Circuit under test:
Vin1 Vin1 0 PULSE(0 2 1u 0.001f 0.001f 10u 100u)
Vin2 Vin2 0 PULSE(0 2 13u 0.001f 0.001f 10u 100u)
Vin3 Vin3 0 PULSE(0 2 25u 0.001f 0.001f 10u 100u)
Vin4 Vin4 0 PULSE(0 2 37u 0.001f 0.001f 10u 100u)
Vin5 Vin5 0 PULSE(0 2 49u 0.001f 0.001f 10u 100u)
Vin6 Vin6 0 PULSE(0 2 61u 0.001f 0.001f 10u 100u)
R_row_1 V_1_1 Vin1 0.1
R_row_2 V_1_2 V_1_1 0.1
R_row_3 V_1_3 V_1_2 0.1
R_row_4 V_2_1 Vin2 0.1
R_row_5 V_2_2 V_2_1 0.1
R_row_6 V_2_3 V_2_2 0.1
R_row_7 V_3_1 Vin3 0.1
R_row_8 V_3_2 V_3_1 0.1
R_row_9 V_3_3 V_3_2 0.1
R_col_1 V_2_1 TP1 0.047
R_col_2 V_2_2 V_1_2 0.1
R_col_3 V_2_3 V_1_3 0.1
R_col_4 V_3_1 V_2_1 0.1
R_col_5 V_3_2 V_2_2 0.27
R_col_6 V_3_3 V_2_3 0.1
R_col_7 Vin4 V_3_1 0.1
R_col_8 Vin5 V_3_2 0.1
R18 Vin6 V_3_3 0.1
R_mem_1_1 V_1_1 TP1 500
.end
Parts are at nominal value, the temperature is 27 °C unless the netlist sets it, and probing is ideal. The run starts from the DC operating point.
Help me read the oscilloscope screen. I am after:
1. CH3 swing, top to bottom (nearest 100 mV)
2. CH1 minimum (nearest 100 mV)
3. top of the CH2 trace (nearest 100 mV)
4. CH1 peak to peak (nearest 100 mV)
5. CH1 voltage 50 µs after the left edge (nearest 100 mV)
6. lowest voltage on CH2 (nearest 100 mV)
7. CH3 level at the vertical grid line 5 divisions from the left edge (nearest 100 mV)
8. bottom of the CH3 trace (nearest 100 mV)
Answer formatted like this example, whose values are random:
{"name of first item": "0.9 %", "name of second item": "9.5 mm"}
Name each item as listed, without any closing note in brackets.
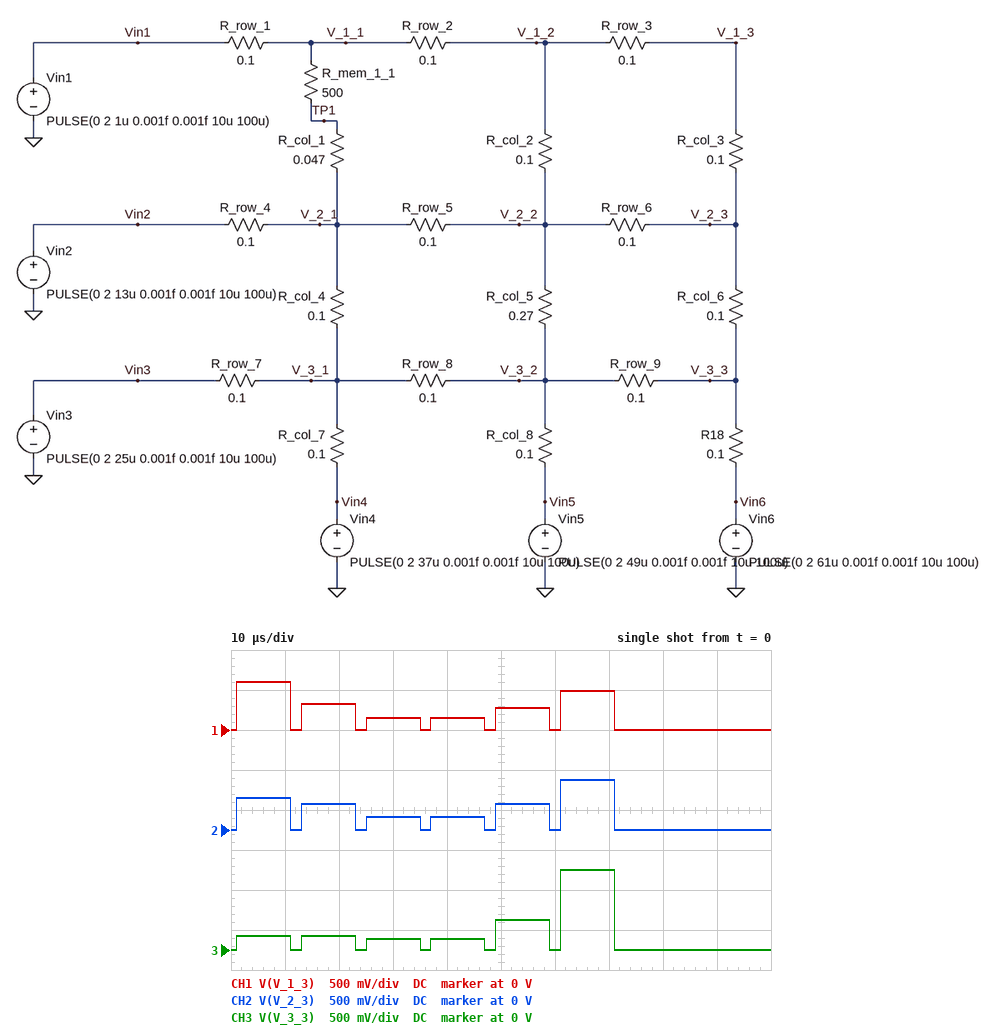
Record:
{"CH3 swing, top to bottom": "1.0 V", "CH1 minimum": "0 V", "top of the CH2 trace": "600 mV", "CH1 peak to peak": "600 mV", "CH1 voltage 50 µs after the left edge": "300 mV", "lowest voltage on CH2": "0 V", "CH3 level at the vertical grid line 5 divisions from the left edge": "400 mV", "bottom of the CH3 trace": "0 V"}
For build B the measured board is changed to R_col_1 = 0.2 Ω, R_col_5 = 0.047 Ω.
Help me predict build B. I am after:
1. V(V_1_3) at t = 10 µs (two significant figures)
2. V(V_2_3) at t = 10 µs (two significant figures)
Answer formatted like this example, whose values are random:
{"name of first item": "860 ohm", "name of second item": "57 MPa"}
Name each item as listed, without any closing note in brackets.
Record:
{"V(V_1_3) at t = 10 µs": "540 mV", "V(V_2_3) at t = 10 µs": "340 mV"}
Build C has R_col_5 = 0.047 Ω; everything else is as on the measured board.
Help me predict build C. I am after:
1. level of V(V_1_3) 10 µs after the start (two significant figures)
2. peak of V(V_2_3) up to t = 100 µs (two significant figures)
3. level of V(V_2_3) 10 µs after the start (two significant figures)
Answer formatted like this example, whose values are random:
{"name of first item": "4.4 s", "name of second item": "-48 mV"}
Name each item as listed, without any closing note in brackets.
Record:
{"level of V(V_1_3) 10 µs after the start": "540 mV", "peak of V(V_2_3) up to t = 100 µs": "620 mV", "level of V(V_2_3) 10 µs after the start": "340 mV"}
